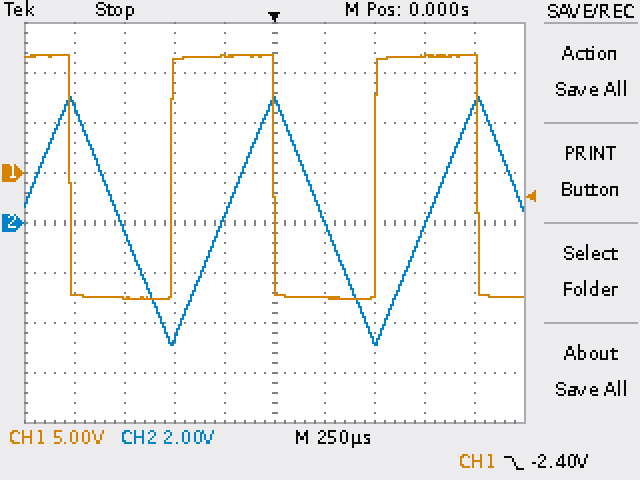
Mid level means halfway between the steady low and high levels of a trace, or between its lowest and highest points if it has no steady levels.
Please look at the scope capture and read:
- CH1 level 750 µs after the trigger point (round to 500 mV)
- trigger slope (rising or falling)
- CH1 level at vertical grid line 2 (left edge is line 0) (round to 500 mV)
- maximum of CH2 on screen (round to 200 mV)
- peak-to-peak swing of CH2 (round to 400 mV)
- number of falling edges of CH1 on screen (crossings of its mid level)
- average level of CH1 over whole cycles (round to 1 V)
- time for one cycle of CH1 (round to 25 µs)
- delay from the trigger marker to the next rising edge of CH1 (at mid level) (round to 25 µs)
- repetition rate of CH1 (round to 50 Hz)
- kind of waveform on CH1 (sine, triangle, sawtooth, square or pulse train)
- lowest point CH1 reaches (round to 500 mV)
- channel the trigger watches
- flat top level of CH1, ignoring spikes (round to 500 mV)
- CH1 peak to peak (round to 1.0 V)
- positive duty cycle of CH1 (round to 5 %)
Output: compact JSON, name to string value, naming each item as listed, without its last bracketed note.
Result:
{"CH1 level 750 µs after the trigger point": "11.5 V", "trigger slope": "falling", "CH1 level at vertical grid line 2 (left edge is line 0)": "-12.5 V", "maximum of CH2 on screen": "5.0 V", "peak-to-peak swing of CH2": "10.0 V", "number of falling edges of CH1 on screen": "3", "average level of CH1 over whole cycles": "0 V", "time for one cycle of CH1": "1.025 ms", "delay from the trigger marker to the next rising edge of CH1 (at mid level)": "500 µs", "repetition rate of CH1": "1.00 kHz", "kind of waveform on CH1": "square", "lowest point CH1 reaches": "-12.5 V", "channel the trigger watches": "CH1", "flat top level of CH1, ignoring spikes": "11.5 V", "CH1 peak to peak": "24.0 V", "positive duty cycle of CH1": "50 %"}
